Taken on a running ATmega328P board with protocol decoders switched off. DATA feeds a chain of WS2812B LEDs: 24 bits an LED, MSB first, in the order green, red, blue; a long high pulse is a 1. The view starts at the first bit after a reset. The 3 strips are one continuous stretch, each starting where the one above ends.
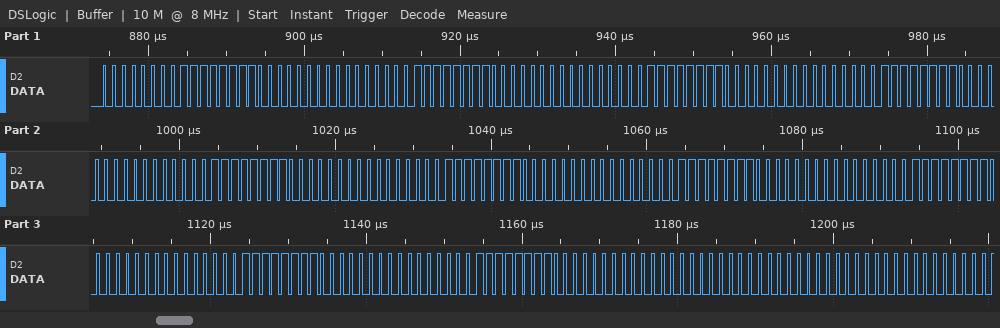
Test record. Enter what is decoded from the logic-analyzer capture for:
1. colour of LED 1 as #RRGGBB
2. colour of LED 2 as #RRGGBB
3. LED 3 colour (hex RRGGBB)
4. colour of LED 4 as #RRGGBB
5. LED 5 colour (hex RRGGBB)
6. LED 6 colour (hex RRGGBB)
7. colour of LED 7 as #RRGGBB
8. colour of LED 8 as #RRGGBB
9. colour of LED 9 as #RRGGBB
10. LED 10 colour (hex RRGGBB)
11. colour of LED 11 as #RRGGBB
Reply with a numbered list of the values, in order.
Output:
1. #FF0000
2. #FF0000
3. #FF0000
4. #FF0000
5. #FF0000
6. #FF0000
7. #FF0000
8. #FF0000
9. #FF0000
10. #FF0000
11. #000000
